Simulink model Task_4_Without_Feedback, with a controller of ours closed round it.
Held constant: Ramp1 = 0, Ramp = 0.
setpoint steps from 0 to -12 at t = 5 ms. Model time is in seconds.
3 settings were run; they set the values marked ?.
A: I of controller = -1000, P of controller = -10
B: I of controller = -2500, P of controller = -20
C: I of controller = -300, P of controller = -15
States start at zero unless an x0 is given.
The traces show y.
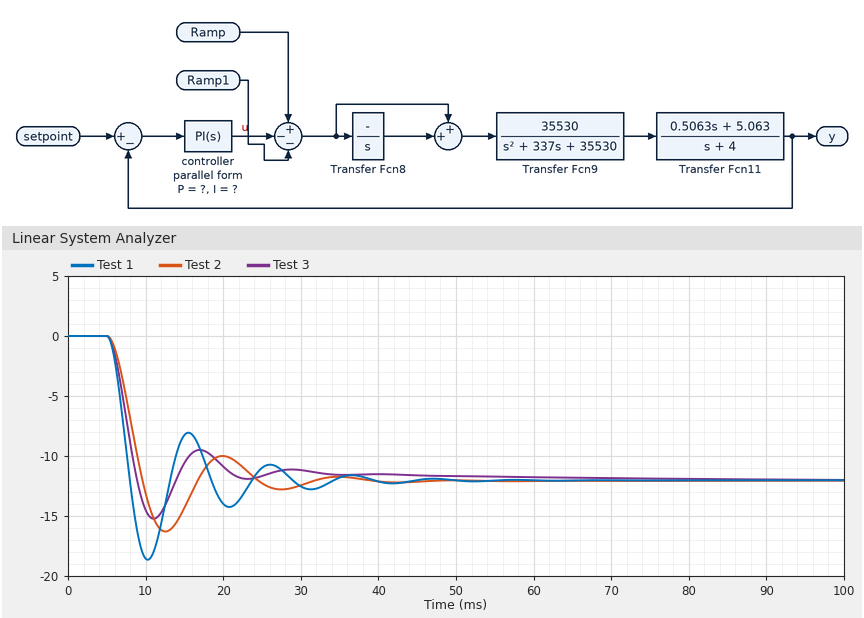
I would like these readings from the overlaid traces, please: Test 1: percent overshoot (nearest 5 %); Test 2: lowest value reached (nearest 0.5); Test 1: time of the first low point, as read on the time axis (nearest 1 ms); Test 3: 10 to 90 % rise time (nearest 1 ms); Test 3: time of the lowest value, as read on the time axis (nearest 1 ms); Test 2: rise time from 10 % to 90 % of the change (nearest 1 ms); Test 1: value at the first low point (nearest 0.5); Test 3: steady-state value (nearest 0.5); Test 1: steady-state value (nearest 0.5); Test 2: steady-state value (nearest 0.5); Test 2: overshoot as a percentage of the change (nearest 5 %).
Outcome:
55 %
-16.5
10 ms
3 ms
11 ms
3 ms
-18.5
-12.0
-12.0
-12.0
35 %
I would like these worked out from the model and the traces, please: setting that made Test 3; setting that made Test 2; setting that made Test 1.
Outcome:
C
A
B
